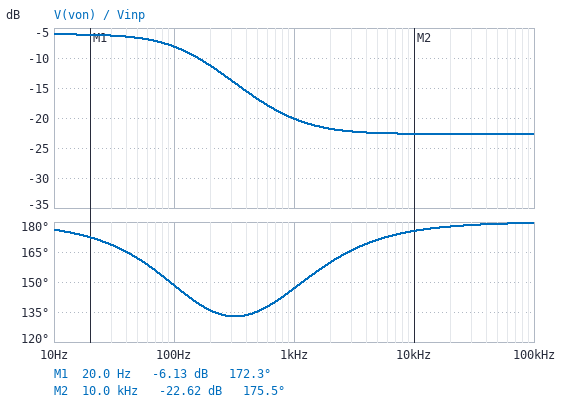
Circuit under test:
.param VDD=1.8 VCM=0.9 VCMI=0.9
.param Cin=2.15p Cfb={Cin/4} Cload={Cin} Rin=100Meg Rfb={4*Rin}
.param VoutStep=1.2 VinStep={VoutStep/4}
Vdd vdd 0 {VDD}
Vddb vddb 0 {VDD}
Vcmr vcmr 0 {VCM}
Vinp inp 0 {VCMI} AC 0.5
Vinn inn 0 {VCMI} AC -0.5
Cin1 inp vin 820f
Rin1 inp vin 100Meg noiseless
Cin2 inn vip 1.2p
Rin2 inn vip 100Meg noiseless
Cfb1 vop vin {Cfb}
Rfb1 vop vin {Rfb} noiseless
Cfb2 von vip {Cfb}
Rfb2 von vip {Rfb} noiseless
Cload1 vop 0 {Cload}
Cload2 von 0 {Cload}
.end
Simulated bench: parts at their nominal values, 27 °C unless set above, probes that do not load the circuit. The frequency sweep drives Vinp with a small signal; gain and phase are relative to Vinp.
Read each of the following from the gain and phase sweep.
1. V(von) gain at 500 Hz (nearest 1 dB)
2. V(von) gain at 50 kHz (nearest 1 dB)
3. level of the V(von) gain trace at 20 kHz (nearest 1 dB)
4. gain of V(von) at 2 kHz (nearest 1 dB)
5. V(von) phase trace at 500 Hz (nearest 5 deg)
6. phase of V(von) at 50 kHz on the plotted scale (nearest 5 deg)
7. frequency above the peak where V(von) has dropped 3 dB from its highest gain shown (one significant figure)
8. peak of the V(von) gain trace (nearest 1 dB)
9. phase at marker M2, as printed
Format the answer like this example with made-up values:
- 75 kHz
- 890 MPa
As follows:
- -17 dB
- -23 dB
- -23 dB
- -22 dB
- 135 deg
- 180 deg
- 100 Hz
- -6 dB
- 175.5 deg
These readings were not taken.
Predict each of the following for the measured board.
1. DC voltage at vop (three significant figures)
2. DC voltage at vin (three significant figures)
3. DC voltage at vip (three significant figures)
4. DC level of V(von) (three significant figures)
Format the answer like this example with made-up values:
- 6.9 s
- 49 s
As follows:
- 900 mV
- 900 mV
- 900 mV
- 900 mV
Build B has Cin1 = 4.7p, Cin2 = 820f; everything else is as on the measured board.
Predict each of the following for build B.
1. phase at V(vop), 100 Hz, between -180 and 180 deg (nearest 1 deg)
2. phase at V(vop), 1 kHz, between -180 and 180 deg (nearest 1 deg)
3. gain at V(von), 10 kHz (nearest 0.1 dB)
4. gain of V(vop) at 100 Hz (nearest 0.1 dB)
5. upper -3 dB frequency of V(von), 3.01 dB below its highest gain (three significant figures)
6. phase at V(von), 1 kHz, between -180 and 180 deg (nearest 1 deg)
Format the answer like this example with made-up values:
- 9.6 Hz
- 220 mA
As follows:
- -31 deg
- -27 deg
- -23.6 dB
- -2.2 dB
- 129 Hz
- 144 deg
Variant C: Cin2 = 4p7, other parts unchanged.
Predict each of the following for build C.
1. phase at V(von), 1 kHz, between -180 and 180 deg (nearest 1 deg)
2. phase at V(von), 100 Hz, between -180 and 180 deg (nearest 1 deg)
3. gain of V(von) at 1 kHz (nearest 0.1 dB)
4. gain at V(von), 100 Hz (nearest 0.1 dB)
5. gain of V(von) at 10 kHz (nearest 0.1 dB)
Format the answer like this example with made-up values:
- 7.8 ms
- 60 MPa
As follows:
- 153 deg
- 149 deg
- -19.1 dB
- -8.2 dB
- -20.7 dB
